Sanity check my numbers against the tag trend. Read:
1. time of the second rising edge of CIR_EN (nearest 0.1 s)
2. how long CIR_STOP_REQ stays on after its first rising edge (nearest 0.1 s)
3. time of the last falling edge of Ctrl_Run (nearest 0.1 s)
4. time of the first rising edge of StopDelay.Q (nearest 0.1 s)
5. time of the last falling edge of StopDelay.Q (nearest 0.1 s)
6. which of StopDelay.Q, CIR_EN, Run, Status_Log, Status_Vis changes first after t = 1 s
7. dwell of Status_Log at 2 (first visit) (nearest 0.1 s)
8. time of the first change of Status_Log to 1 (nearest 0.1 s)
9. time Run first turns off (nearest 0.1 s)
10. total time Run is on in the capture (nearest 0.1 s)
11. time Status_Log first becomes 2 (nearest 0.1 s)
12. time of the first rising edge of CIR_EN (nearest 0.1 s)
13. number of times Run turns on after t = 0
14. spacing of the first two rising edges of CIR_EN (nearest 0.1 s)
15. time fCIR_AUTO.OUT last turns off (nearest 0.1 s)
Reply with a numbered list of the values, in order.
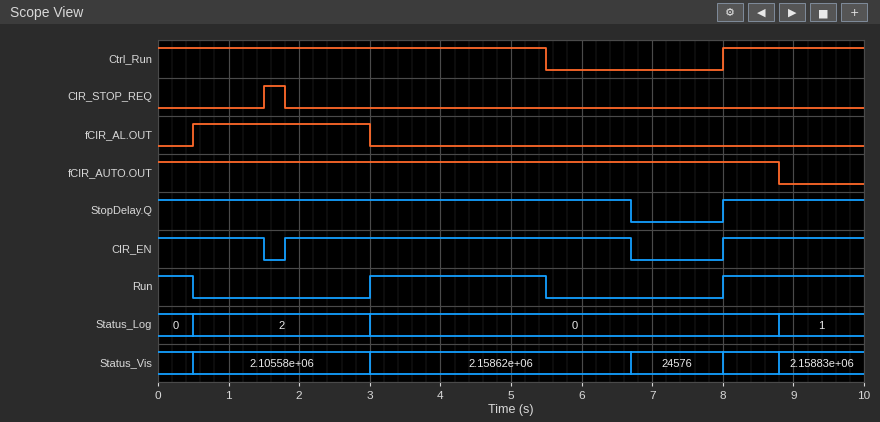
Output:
1. 8.0 s
2. 0.3 s
3. 5.5 s
4. 8.0 s
5. 6.7 s
6. CIR_EN
7. 2.5 s
8. 8.8 s
9. 0.5 s
10. 5.0 s
11. 0.5 s
12. 1.8 s
13. 2
14. 6.2 s
15. 8.8 s
